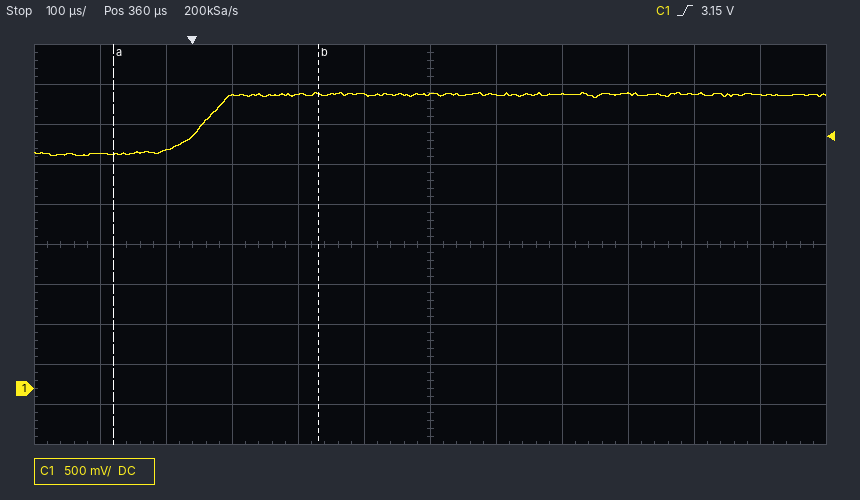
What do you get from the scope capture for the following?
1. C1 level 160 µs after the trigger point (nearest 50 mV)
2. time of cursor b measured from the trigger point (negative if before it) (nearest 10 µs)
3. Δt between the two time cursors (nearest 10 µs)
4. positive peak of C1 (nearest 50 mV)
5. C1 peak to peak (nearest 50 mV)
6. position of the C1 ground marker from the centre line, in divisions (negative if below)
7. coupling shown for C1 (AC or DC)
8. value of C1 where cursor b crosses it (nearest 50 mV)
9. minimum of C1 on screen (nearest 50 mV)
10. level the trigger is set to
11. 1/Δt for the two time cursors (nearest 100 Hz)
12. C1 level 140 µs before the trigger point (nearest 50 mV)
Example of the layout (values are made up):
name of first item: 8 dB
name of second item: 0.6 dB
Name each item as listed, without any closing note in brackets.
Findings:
C1 level 160 µs after the trigger point: 3.70 V
time of cursor b measured from the trigger point (negative if before it): +190 µs
Δt between the two time cursors: 310 µs
positive peak of C1: 3.70 V
C1 peak to peak: 800 mV
position of the C1 ground marker from the centre line, in divisions: -3.6 div
coupling shown for C1: DC
value of C1 where cursor b crosses it: 3.70 V
minimum of C1 on screen: 2.90 V
level the trigger is set to: 3.15 V
1/Δt for the two time cursors: 3.2 kHz
C1 level 140 µs before the trigger point: 2.95 V
